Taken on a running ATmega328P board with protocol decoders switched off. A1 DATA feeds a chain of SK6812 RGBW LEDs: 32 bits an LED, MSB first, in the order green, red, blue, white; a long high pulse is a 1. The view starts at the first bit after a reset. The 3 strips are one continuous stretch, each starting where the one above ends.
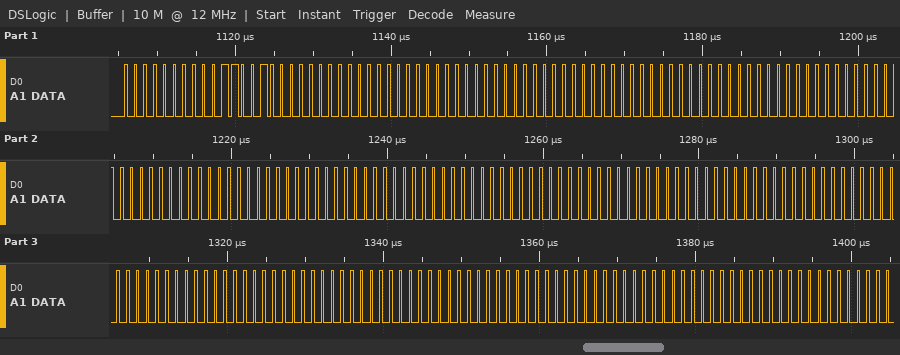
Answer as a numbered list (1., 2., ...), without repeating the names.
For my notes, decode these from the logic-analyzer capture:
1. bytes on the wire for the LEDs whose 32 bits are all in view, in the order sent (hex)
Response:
1. 00 32 00 00 00 00 00 00 00 00 00 00 00 00 00 00 00 00 00 00 00 00 00 00 00 00 00 00
